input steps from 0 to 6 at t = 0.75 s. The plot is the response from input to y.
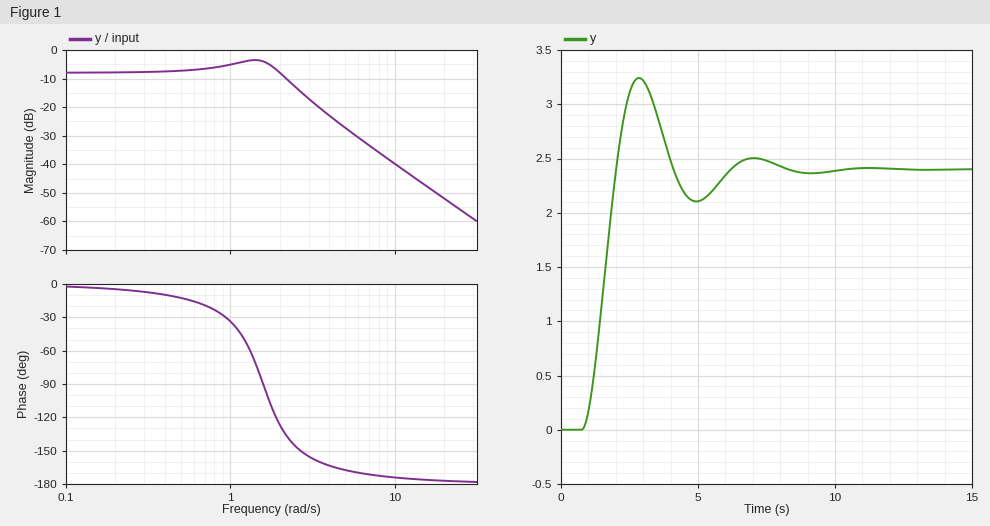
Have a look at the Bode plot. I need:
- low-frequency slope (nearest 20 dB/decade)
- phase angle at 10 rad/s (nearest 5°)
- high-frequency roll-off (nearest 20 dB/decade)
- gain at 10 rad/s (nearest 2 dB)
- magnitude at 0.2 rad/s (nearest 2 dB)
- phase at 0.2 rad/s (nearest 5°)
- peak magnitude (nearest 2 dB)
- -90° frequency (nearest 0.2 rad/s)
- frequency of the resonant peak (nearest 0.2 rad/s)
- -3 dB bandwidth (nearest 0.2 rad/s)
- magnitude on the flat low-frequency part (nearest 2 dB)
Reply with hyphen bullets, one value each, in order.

- 0 dB/decade
- -175°
- -40 dB/decade
- -40 dB
- -8 dB
- -5°
- -4 dB
- 1.6 rad/s
- 1.4 rad/s
- 2.2 rad/s
- -8 dB
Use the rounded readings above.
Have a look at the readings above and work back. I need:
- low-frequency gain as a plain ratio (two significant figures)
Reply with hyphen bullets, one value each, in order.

- 0.40
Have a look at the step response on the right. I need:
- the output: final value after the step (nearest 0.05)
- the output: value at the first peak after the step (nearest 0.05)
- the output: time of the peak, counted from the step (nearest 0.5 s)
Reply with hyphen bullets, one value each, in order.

- 2.40
- 3.25
- 2.0 s
